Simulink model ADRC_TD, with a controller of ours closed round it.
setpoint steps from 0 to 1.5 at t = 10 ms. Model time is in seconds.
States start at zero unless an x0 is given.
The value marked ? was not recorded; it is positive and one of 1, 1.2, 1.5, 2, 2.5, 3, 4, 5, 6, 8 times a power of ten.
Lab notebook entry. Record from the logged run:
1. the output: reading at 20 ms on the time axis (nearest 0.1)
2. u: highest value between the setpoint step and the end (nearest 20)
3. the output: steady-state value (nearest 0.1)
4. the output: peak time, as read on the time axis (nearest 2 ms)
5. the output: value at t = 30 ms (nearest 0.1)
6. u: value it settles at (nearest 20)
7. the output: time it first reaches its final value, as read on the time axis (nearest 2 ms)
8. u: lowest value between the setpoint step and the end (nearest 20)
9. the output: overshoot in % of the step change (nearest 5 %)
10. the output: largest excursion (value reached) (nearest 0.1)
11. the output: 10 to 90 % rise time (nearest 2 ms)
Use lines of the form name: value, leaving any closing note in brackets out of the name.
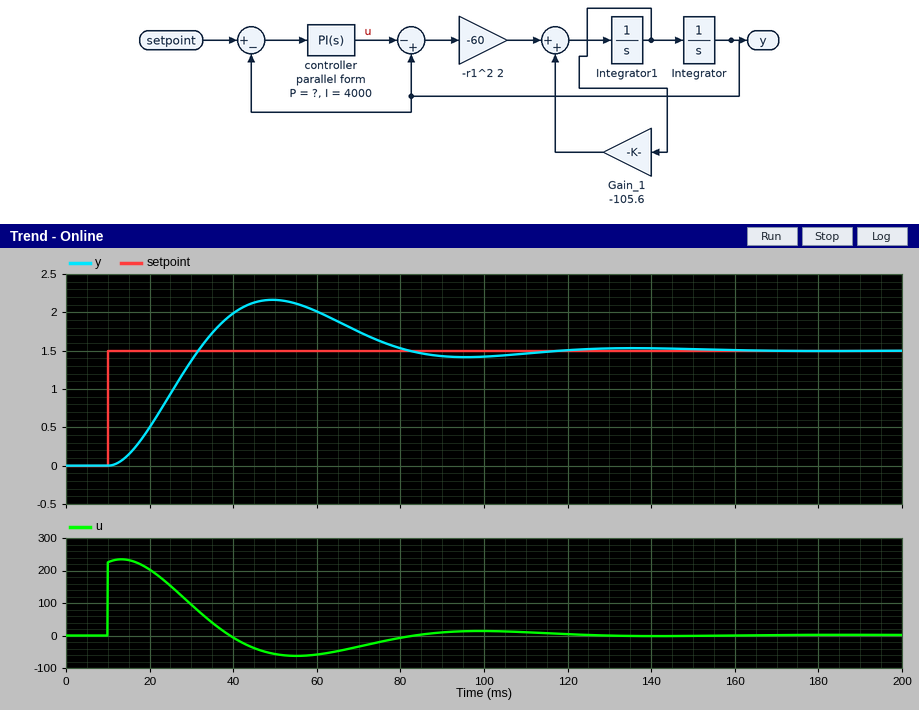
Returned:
the output: reading at 20 ms on the time axis: 0.5
u: highest value between the setpoint step and the end: 240
the output: steady-state value: 1.5
the output: peak time, as read on the time axis: 50 ms
the output: value at t = 30 ms: 1.4
u: value it settles at: 0
the output: time it first reaches its final value, as read on the time axis: 32 ms
u: lowest value between the setpoint step and the end: -60
the output: overshoot in % of the step change: 45 %
the output: largest excursion (value reached): 2.2
the output: 10 to 90 % rise time: 14 ms
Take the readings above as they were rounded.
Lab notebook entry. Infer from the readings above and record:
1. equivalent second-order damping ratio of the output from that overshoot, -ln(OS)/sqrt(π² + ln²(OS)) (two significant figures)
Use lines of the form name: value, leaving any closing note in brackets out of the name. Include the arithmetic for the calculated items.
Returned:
equivalent second-order damping ratio of the output from that overshoot, -ln(OS)/sqrt(π² + ln²(OS)): ln(0.45) = -0.799; 0.799 / sqrt(9.870 + 0.638) = 0.25
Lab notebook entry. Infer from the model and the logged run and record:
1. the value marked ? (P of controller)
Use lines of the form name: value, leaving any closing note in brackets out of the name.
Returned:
the value marked ?: 150
